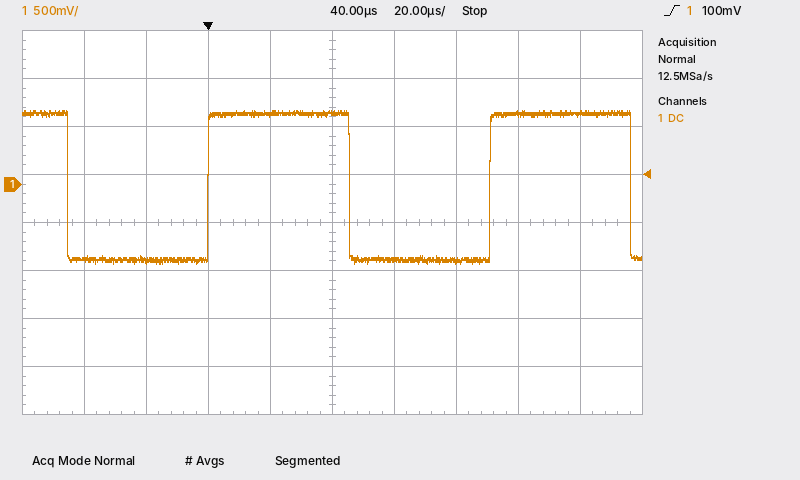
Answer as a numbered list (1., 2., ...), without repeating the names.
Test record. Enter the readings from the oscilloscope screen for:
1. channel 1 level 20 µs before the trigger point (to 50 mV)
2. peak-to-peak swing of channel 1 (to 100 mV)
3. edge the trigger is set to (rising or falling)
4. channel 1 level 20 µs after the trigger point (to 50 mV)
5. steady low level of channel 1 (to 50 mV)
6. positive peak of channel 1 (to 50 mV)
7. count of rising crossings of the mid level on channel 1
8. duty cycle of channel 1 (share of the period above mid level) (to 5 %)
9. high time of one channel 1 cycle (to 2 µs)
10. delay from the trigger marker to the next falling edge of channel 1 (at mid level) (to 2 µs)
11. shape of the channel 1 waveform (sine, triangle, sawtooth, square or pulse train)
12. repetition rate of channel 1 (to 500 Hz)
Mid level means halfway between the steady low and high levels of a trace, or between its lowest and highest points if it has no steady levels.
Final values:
1. -800 mV
2. 1.60 V
3. rising
4. 750 mV
5. -800 mV
6. 750 mV
7. 2
8. 50 %
9. 46 µs
10. 46 µs
11. square
12. 11.0 kHz
